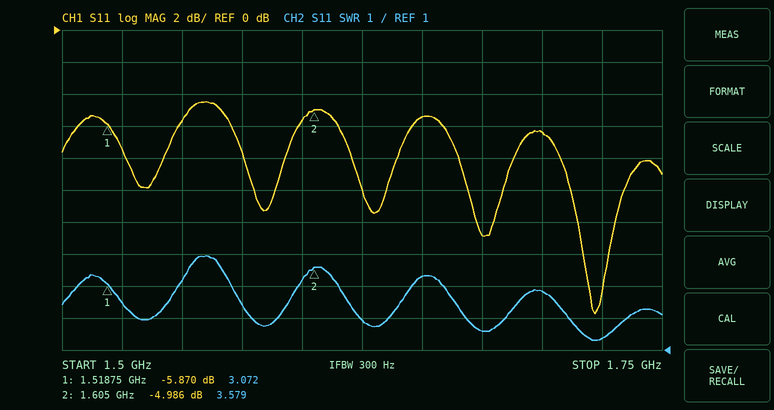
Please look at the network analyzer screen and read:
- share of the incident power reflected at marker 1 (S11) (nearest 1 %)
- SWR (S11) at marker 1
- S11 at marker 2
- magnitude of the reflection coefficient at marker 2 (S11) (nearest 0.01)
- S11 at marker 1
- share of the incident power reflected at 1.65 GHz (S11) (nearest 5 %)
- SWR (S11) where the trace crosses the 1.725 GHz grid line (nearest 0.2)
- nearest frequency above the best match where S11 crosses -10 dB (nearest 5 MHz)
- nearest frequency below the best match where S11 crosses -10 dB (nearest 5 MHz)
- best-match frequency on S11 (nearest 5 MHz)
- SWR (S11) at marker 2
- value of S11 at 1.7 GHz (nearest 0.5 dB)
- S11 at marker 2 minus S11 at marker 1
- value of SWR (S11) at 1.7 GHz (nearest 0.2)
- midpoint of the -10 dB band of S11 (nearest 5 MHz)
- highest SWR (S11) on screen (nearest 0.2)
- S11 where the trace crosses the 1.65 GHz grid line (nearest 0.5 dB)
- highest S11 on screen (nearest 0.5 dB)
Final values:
26 %
3.072
-4.986 dB
0.56
-5.870 dB
30 %
1.4
1.735 GHz
1.710 GHz
1.720 GHz
3.579
-6.5 dB
0.884 dB
2.8
1.725 GHz
4.0
-5.5 dB
-4.5 dB
